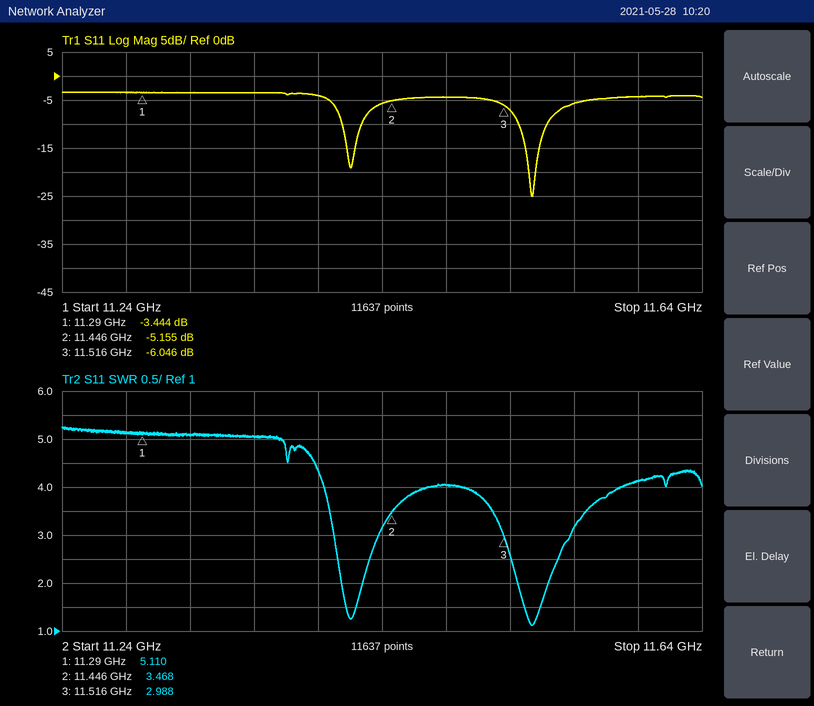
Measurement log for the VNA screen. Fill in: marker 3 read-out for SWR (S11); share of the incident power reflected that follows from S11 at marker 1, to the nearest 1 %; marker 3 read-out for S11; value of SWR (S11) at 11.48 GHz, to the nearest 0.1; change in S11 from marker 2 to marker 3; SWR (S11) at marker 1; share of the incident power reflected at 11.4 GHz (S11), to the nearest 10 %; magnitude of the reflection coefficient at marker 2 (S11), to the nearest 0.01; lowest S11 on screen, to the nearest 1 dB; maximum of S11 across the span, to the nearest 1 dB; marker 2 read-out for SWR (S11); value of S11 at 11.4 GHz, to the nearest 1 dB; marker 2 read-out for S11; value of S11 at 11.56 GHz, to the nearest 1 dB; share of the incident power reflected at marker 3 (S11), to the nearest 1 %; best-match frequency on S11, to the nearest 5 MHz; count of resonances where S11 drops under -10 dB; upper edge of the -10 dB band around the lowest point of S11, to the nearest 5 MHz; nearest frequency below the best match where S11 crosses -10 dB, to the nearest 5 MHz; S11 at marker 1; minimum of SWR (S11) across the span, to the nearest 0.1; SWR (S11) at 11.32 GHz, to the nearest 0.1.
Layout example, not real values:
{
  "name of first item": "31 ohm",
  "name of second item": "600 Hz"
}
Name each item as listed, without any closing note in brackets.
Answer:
{
  "marker 3 read-out for SWR": "2.988",
  "share of the incident power reflected that follows from S11 at marker 1, to the nearest 1 %": "45 %",
  "marker 3 read-out for S11": "-6.046 dB",
  "value of SWR (S11) at 11.48 GHz, to the nearest 0.1": "4.0",
  "change in S11 from marker 2 to marker 3": "-0.891 dB",
  "SWR (S11) at marker 1": "5.110",
  "share of the incident power reflected at 11.4 GHz (S11), to the nearest 10 %": "40 %",
  "magnitude of the reflection coefficient at marker 2 (S11), to the nearest 0.01": "0.55",
  "lowest S11 on screen, to the nearest 1 dB": "-25 dB",
  "maximum of S11 across the span, to the nearest 1 dB": "-3 dB",
  "marker 2 read-out for SWR": "3.468",
  "value of S11 at 11.4 GHz, to the nearest 1 dB": "-4 dB",
  "marker 2 read-out for S11": "-5.155 dB",
  "value of S11 at 11.56 GHz, to the nearest 1 dB": "-6 dB",
  "share of the incident power reflected at marker 3 (S11), to the nearest 1 %": "25 %",
  "best-match frequency on S11, to the nearest 5 MHz": "11.535 GHz",
  "count of resonances where S11 drops under -10 dB": "2",
  "upper edge of the -10 dB band around the lowest point of S11, to the nearest 5 MHz": "11.545 GHz",
  "nearest frequency below the best match where S11 crosses -10 dB, to the nearest 5 MHz": "11.525 GHz",
  "S11 at marker 1": "-3.444 dB",
  "minimum of SWR (S11) across the span, to the nearest 0.1": "1.1",
  "SWR (S11) at 11.32 GHz, to the nearest 0.1": "5.1"
}
